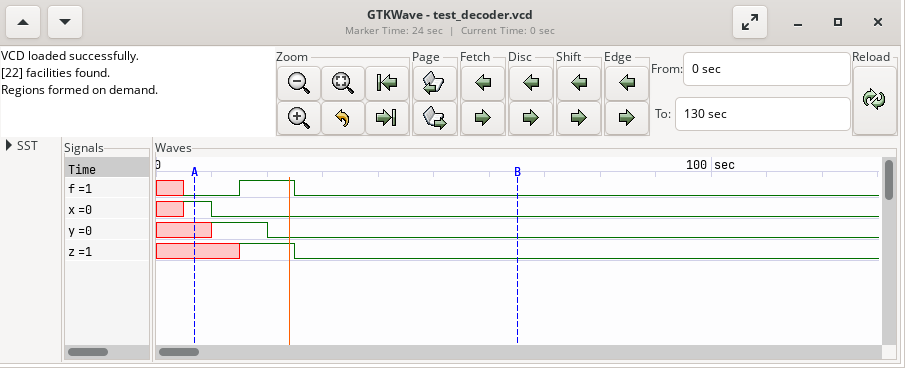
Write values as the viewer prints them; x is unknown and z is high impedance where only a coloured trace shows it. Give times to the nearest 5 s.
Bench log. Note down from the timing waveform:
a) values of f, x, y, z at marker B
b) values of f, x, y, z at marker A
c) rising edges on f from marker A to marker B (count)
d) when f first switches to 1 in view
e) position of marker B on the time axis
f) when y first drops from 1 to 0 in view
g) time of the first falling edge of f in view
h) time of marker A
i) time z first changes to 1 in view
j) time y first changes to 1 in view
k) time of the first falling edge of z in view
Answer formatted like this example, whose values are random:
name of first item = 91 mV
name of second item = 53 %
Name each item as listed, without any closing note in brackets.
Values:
values of f, x, y, z at marker B = f=0, x=0, y=0, z=0
values of f, x, y, z at marker A = f=0, x=1, y=x, z=x
rising edges on f from marker A to marker B = 1
when f first switches to 1 in view = 15 s
position of marker B on the time axis = 65 s
when y first drops from 1 to 0 in view = 20 s
time of the first falling edge of f in view = 25 s
time of marker A = 5 s
time z first changes to 1 in view = 15 s
time y first changes to 1 in view = 10 s
time of the first falling edge of z in view = 25 s
